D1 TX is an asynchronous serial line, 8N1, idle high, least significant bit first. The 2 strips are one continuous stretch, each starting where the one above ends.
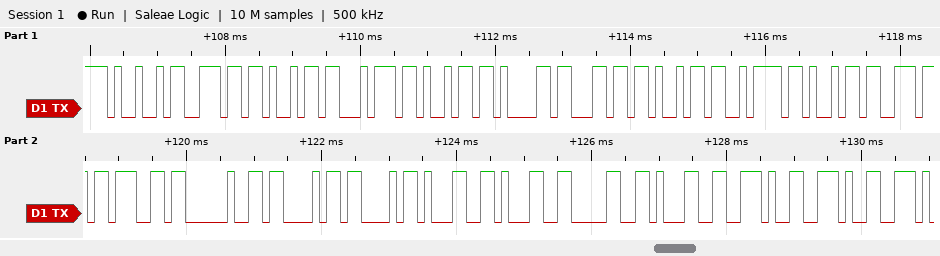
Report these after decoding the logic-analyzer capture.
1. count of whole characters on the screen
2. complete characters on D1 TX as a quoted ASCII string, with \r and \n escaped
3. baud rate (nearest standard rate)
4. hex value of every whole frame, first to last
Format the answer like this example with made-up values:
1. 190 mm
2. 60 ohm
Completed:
1. 21
2. "Initializing CC1101.."
3. 9600 baud
4. 0x49 0x6E 0x69 0x74 0x69 0x61 0x6C 0x69 0x7A 0x69 0x6E 0x67 0x20 0x43 0x43 0x31 0x31 0x30 0x31 0x2E 0x2E
